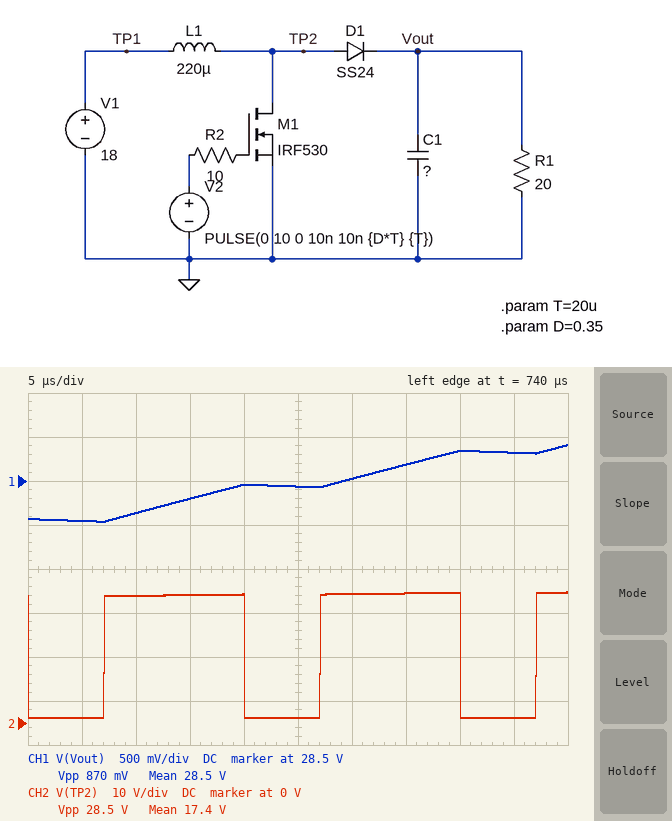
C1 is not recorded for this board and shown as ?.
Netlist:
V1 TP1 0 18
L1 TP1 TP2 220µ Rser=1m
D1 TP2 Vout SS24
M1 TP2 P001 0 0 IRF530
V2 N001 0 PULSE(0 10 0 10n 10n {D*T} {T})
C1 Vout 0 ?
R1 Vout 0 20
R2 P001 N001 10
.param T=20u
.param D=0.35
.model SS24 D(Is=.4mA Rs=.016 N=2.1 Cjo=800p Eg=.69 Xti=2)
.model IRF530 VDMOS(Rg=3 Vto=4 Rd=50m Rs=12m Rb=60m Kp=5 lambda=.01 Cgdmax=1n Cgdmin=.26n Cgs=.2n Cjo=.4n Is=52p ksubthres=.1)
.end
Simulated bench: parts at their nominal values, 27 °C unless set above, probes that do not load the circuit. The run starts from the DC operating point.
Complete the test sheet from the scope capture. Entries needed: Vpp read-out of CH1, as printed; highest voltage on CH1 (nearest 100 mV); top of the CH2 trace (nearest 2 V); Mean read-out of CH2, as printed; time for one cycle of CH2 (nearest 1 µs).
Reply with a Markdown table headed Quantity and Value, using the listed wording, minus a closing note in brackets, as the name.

| Quantity | Value |
|---|---|
| Vpp read-out of CH1, as printed | 870 mV |
| highest voltage on CH1 | 28.9 V |
| top of the CH2 trace | 30 V |
| Mean read-out of CH2, as printed | 17.4 V |
| time for one cycle of CH2 | 20 µs |
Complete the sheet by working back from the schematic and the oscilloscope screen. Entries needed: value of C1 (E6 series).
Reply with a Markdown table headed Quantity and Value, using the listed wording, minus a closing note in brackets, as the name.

| Quantity | Value |
|---|---|
| value of C1 | 330 µF |
